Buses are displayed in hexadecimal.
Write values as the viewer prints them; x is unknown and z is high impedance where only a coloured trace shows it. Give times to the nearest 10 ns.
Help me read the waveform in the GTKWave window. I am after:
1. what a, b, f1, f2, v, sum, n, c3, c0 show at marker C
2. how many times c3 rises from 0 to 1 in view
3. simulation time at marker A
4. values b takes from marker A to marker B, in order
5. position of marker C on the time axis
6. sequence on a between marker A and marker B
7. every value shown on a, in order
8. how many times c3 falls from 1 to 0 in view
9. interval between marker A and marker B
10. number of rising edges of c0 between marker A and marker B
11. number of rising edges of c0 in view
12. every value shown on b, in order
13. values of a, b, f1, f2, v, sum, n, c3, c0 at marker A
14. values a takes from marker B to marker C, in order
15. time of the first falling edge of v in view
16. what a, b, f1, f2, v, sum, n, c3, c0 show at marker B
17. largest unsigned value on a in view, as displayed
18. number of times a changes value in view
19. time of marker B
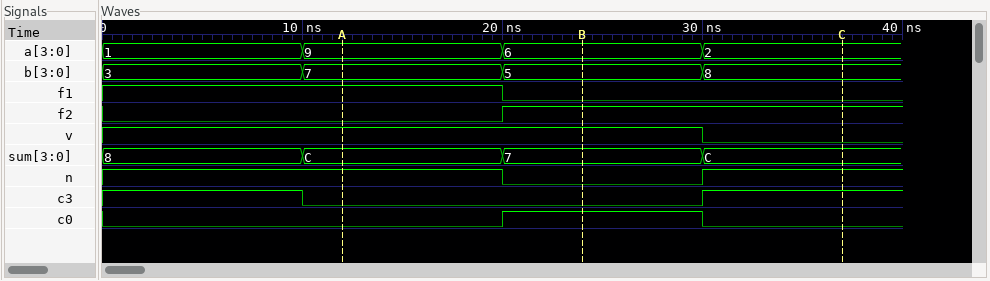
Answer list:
a=2, b=8, f1=0, f2=1, v=0, sum=C, n=1, c3=1, c0=0
1
10 ns
7, 5
40 ns
9, 6
1, 9, 6, 2
1
10 ns
1
1
3, 7, 5, 8
a=9, b=7, f1=1, f2=0, v=1, sum=C, n=1, c3=0, c0=0
6, 2
30 ns
a=6, b=5, f1=0, f2=1, v=1, sum=7, n=0, c3=0, c0=1
9
3
20 ns
